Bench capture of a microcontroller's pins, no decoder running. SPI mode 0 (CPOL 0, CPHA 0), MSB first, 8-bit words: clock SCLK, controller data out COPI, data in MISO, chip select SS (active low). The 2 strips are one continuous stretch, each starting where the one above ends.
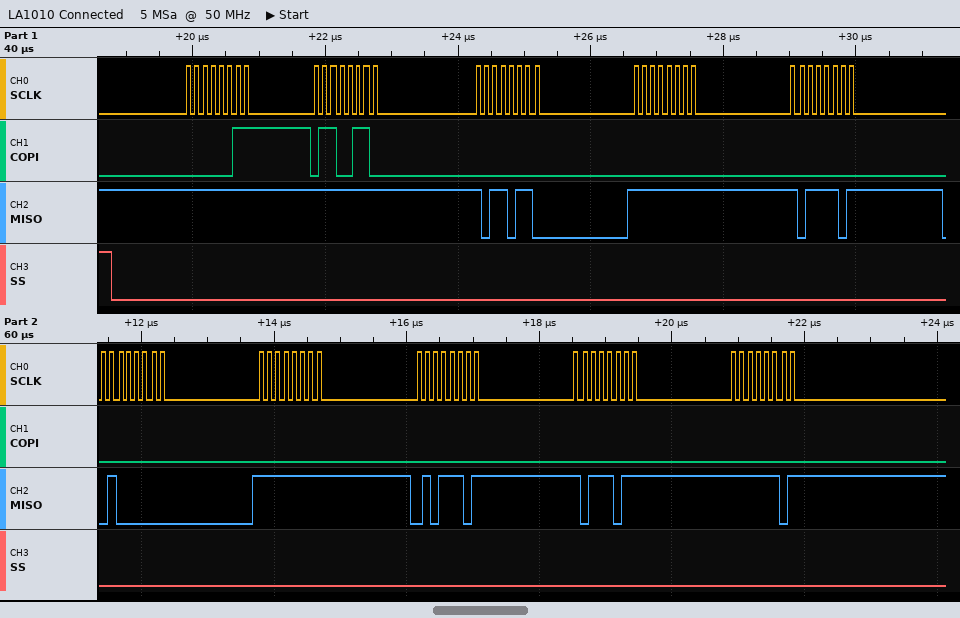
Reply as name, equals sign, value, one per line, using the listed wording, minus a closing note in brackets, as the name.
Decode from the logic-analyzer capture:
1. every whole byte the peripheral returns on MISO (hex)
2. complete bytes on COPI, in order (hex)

every whole byte the peripheral returns on MISO = FF FF B6 FF BD 40 FF 5D BB FD
complete bytes on COPI, in order = 03 66 00 00 00 00 00 00 00 00
